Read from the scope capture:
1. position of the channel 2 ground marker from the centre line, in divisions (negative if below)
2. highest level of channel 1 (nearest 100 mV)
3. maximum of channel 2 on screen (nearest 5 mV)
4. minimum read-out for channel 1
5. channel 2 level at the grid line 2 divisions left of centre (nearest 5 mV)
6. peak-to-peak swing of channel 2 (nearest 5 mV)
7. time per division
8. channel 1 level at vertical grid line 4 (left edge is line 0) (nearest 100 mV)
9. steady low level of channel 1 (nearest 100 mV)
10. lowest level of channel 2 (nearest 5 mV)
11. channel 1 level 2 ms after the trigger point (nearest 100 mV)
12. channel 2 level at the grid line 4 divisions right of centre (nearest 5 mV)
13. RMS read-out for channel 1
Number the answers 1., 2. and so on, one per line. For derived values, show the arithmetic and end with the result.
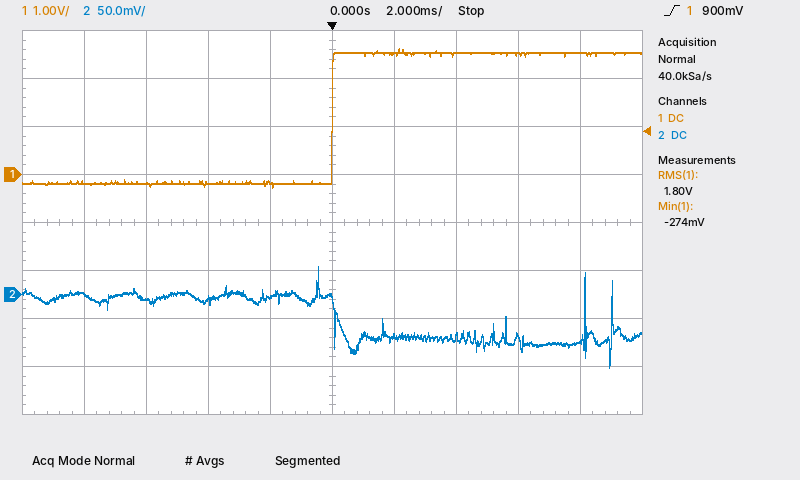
1. -1.5 div
2. 2.6 V
3. 30 mV
4. -274 mV
5. -5 mV
6. 30 mV − (-75 mV) = 105 mV
7. 2 ms
8. -200 mV
9. -200 mV
10. -75 mV
11. 2.5 V
12. -45 mV
13. 1.80 V
